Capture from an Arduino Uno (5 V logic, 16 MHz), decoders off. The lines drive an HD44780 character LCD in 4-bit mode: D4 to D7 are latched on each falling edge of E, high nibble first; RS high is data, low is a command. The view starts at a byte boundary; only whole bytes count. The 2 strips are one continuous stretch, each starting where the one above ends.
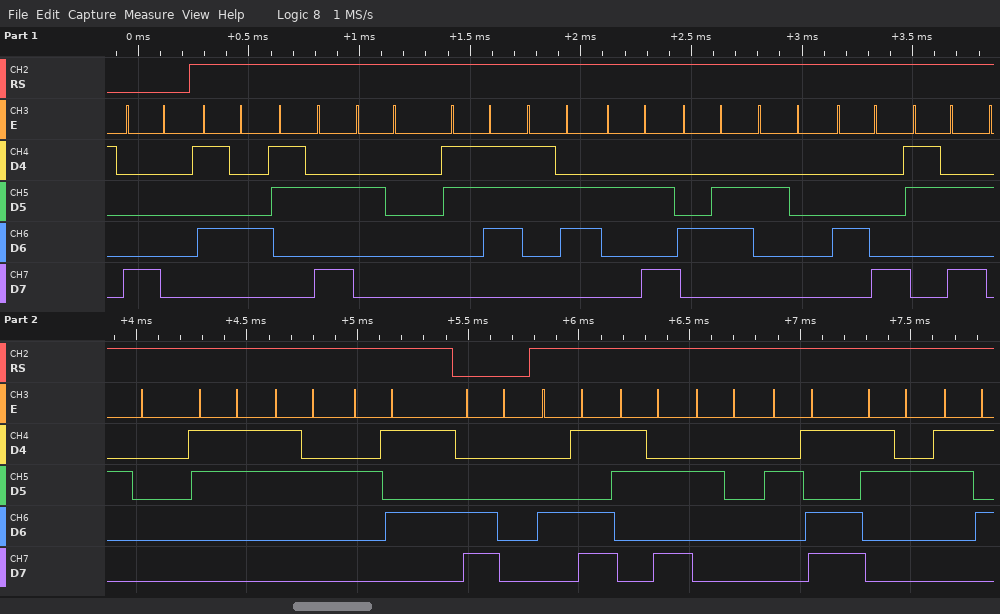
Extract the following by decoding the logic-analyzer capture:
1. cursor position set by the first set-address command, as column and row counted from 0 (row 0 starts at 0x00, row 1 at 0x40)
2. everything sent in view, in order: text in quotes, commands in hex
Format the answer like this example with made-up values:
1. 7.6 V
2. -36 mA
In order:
1. column 0, row 0
2. 0x80 "T: 76*F H: 32%" 0xC0 "M: -25"
